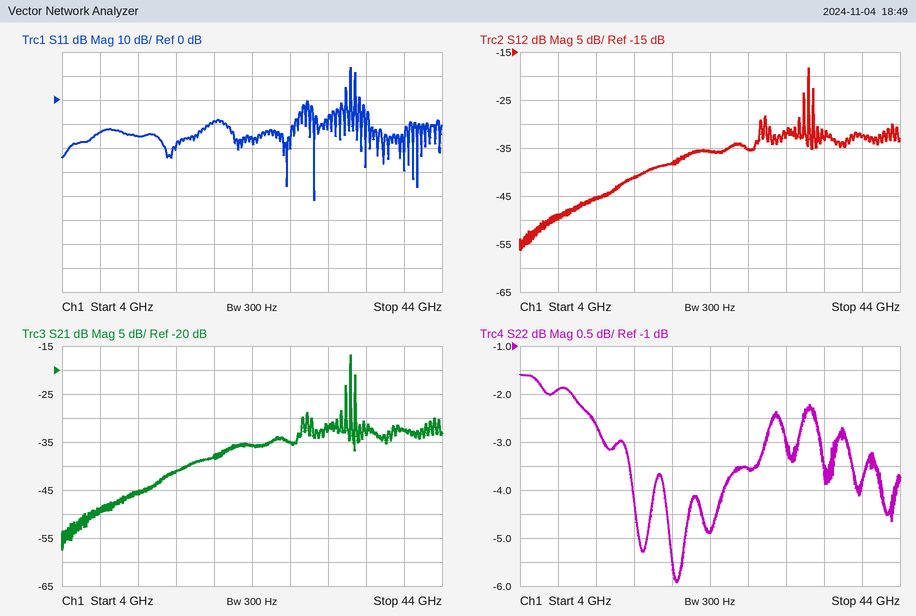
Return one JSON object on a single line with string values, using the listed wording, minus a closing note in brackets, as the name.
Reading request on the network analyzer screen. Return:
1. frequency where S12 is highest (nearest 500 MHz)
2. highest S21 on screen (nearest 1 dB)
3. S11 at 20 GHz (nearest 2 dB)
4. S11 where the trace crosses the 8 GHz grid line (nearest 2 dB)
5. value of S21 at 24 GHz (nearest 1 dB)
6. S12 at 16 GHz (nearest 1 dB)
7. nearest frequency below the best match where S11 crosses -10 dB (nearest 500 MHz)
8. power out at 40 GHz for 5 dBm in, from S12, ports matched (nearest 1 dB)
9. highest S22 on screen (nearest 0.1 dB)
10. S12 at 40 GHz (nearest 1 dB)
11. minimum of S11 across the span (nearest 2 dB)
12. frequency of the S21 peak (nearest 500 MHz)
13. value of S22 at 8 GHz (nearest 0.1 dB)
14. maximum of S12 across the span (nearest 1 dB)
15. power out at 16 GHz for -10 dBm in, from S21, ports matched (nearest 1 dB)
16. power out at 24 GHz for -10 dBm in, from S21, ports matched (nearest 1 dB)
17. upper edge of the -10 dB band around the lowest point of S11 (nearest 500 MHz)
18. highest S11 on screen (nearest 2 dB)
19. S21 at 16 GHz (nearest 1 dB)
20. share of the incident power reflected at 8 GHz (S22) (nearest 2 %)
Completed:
{"frequency where S12 is highest": "34.5 GHz", "highest S21 on screen": "-17 dB", "S11 at 20 GHz": "-8 dB", "S11 where the trace crosses the 8 GHz grid line": "-14 dB", "value of S21 at 24 GHz": "-36 dB", "S12 at 16 GHz": "-41 dB", "nearest frequency below the best match where S11 crosses -10 dB": "30.5 GHz", "power out at 40 GHz for 5 dBm in, from S12, ports matched": "-28 dBm", "highest S22 on screen": "-1.6 dB", "S12 at 40 GHz": "-33 dB", "minimum of S11 across the span": "-42 dB", "frequency of the S21 peak": "34.5 GHz", "value of S22 at 8 GHz": "-1.9 dB", "maximum of S12 across the span": "-18 dB", "power out at 16 GHz for -10 dBm in, from S21, ports matched": "-51 dBm", "power out at 24 GHz for -10 dBm in, from S21, ports matched": "-46 dBm", "upper edge of the -10 dB band around the lowest point of S11": "30.5 GHz", "highest S11 on screen": "14 dB", "S21 at 16 GHz": "-41 dB", "share of the incident power reflected at 8 GHz (S22)": "64 %"}
